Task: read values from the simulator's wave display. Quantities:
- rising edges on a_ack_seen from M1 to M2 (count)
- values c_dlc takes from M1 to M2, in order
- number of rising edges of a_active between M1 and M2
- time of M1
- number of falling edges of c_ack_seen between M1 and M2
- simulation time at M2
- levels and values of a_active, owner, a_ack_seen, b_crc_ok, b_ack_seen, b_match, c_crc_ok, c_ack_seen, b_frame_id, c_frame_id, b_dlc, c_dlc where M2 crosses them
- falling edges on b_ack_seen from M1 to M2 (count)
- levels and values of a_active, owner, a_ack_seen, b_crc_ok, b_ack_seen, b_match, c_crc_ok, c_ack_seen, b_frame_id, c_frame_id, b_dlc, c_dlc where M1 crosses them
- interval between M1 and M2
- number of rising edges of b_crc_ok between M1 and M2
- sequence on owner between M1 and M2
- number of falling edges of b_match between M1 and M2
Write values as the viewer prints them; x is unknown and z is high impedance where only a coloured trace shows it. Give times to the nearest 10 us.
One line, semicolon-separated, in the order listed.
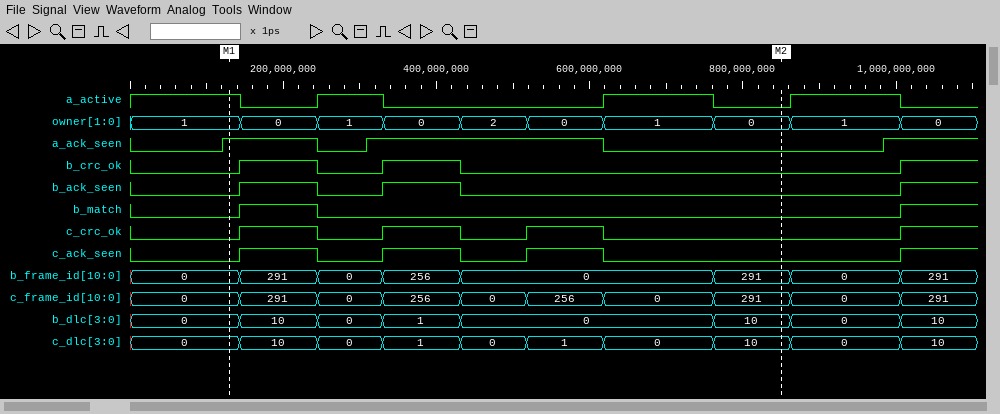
1; 0, 10, 0, 1, 0, 1, 0, 10; 2; 130 us; 3; 850 us; a_active=0, owner=0, a_ack_seen=0, b_crc_ok=0, b_ack_seen=0, b_match=0, c_crc_ok=0, c_ack_seen=0, b_frame_id=291, c_frame_id=291, b_dlc=10, c_dlc=10; 2; a_active=1, owner=1, a_ack_seen=1, b_crc_ok=0, b_ack_seen=0, b_match=0, c_crc_ok=0, c_ack_seen=0, b_frame_id=0, c_frame_id=0, b_dlc=0, c_dlc=0; 720 us; 2; 1, 0, 1, 0, 2, 0, 1, 0; 1
